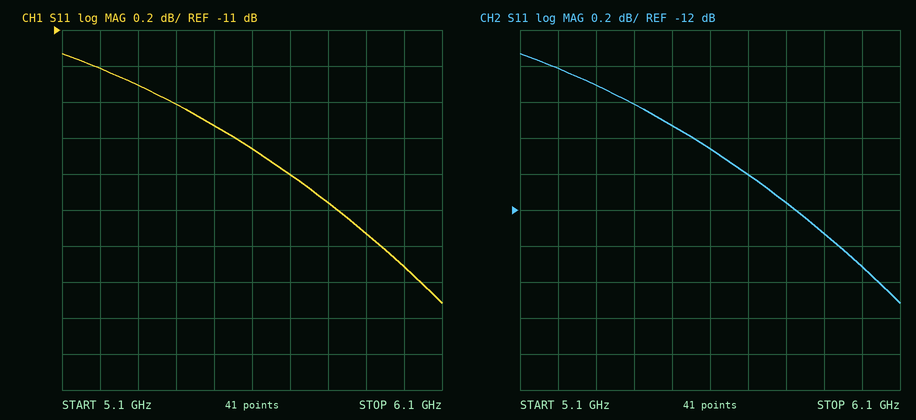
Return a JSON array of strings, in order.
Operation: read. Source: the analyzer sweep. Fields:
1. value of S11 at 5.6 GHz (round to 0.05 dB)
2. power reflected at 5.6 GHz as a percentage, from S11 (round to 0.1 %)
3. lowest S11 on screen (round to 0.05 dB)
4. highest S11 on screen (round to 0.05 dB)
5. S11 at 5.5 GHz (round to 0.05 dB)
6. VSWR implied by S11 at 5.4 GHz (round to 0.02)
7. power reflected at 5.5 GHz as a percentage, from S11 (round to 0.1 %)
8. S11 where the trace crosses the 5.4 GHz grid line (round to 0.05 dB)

["-11.65 dB", "6.8 %", "-12.50 dB", "-11.15 dB", "-11.55 dB", "1.74", "7.0 %", "-11.40 dB"]
